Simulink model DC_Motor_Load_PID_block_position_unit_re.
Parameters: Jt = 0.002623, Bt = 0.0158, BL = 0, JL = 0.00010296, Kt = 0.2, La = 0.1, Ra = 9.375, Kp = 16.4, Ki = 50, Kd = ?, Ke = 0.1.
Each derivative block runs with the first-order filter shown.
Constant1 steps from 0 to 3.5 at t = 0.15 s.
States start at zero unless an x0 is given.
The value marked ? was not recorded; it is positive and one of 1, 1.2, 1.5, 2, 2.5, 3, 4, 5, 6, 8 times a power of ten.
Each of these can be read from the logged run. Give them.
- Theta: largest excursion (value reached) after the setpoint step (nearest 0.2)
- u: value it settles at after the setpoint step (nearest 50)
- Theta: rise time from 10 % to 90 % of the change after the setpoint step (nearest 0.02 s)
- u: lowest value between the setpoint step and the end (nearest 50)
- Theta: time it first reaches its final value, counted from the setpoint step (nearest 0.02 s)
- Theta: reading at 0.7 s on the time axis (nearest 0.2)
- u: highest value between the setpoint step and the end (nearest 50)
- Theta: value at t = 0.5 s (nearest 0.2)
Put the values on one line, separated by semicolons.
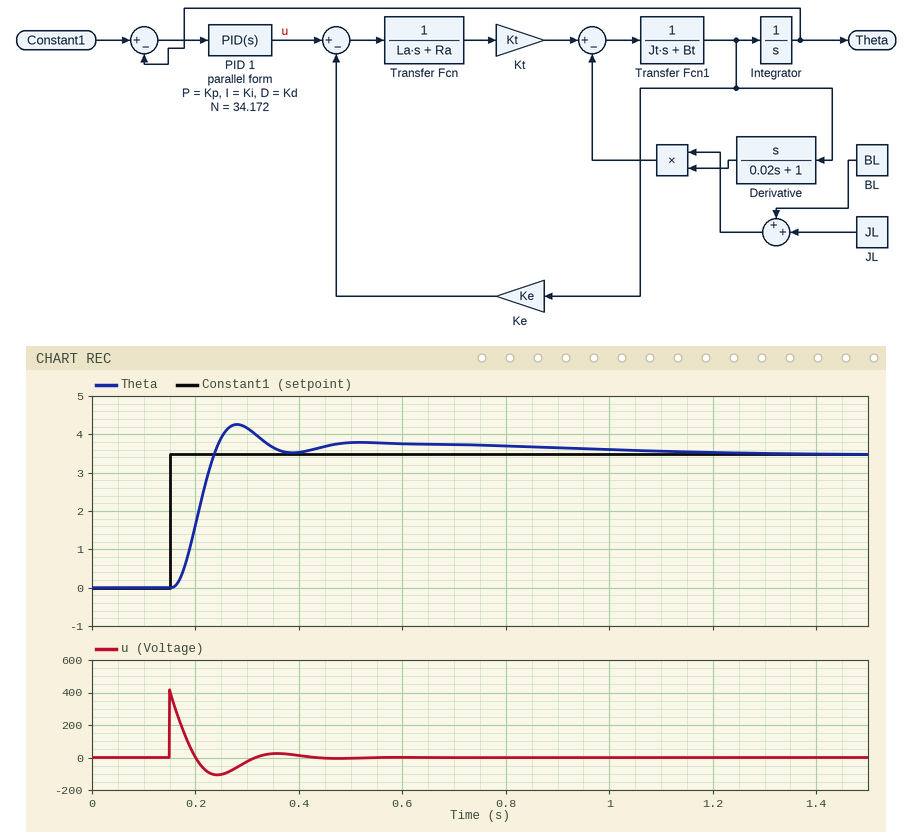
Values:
4.2; 0; 0.06 s; -100; 0.08 s; 3.8; 400; 3.8
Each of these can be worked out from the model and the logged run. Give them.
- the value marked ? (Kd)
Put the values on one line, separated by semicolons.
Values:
3
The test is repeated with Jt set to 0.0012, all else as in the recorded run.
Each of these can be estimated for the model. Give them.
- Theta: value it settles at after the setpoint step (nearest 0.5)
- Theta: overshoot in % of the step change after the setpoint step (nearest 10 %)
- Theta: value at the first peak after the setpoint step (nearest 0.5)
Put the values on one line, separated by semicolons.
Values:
3.5; 30 %; 4.5
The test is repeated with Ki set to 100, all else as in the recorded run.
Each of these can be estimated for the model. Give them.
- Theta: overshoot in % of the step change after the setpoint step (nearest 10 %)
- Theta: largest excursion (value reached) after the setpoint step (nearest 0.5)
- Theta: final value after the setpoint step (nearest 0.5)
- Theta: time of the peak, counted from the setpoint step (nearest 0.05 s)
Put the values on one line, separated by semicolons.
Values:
30 %; 4.5; 3.5; 0.15 s
